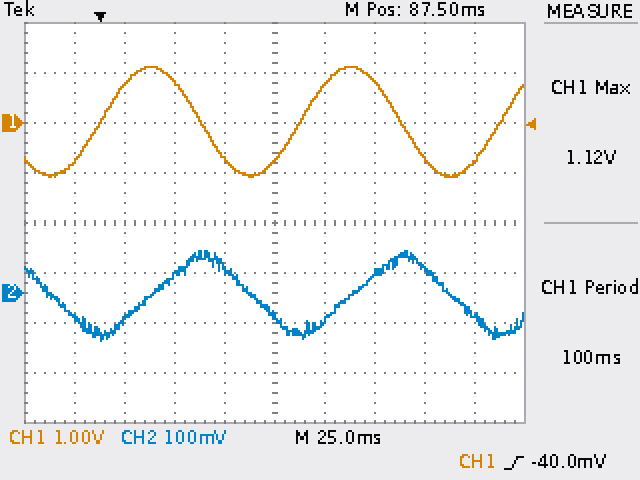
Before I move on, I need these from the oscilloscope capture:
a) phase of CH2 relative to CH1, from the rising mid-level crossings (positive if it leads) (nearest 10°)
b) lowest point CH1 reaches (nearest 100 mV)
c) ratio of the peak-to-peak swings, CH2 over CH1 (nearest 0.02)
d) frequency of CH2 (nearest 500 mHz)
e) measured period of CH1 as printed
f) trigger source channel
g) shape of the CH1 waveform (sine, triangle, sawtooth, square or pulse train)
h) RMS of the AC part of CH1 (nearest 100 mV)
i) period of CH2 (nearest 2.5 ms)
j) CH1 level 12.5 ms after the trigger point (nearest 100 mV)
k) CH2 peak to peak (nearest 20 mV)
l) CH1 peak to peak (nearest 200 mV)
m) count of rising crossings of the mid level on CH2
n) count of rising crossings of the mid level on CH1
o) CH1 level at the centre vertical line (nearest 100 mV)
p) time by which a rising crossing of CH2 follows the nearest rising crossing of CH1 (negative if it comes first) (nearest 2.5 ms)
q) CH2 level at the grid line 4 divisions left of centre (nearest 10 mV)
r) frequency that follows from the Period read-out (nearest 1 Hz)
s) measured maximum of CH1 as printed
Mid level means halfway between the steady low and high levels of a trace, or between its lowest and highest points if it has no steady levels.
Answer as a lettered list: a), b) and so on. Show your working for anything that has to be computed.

a) −360° × (+25.0 ms) / 100.0 ms ≈ -90°
b) -1.1 V
c) 180 mV / 2.2 V ≈ 0.08
d) 1 / 100.0 ms ≈ 10.0 Hz
e) 100 ms
f) CH1
g) sine
h) 2.2 V / (2√2) ≈ 778 mV, so 800 mV to the nearest 100 mV
i) 100.0 ms
j) 800 mV
k) 180 mV
l) 2.2 V
m) 2
n) 3
o) -800 mV
p) +25.0 ms
q) -50 mV
r) 1 / 100 ms ≈ 10 Hz
s) 1.12 V
